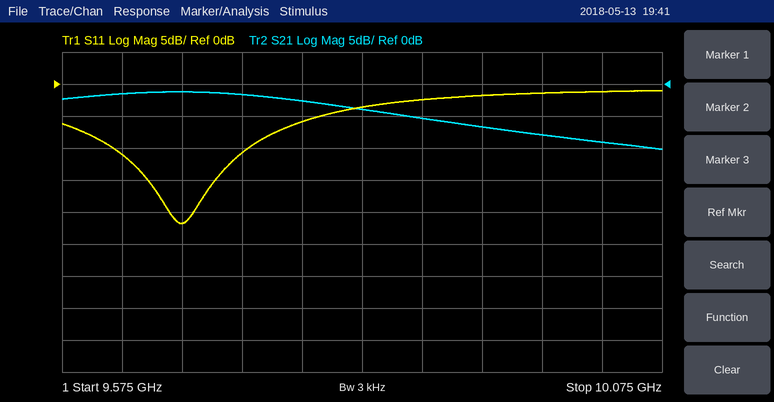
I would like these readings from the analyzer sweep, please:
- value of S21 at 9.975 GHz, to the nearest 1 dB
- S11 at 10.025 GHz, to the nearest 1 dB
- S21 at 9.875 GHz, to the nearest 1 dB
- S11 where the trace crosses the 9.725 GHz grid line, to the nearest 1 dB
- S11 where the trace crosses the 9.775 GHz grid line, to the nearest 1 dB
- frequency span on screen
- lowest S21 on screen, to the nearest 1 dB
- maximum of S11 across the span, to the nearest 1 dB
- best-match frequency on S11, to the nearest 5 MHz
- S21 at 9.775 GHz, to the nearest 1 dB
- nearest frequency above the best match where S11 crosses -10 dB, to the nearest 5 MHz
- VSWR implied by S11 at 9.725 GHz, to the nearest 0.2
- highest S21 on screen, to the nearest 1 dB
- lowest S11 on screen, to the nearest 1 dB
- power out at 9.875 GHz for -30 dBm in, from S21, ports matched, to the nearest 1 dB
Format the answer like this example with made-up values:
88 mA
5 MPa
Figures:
-8 dB
-1 dB
-5 dB
-11 dB
-6 dB
500 MHz
-10 dB
-1 dB
9.675 GHz
-3 dB
9.730 GHz
1.8
-1 dB
-22 dB
-35 dBm
